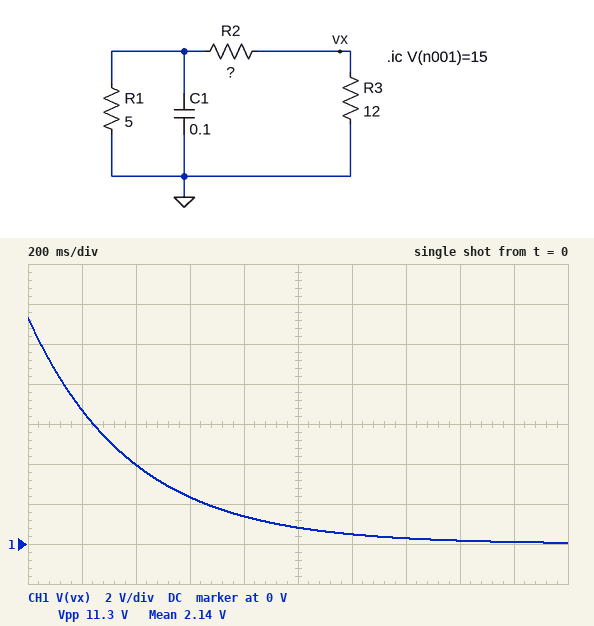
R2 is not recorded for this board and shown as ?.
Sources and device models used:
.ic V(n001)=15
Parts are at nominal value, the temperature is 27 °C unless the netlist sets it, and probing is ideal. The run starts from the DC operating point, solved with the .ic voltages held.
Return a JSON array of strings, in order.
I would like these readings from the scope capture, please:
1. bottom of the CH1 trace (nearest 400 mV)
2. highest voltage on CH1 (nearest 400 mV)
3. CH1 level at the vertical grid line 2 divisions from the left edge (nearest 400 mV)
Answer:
["0 V", "11.2 V", "4.0 V"]
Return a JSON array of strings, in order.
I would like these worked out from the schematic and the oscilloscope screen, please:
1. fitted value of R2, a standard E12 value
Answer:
["3.9 Ω"]
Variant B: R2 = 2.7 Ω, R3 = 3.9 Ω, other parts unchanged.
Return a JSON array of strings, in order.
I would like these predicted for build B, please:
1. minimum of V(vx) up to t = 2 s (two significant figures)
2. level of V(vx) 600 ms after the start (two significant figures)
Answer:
["7.8 mV", "1.1 V"]
